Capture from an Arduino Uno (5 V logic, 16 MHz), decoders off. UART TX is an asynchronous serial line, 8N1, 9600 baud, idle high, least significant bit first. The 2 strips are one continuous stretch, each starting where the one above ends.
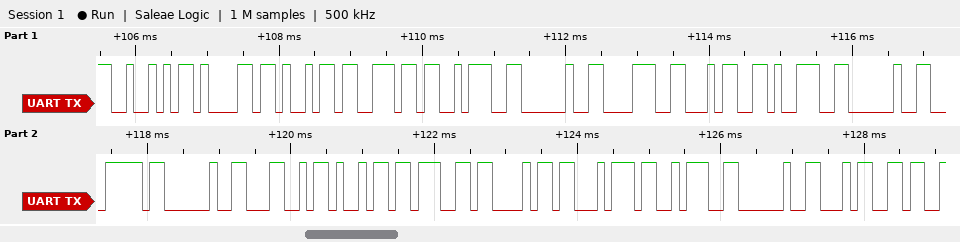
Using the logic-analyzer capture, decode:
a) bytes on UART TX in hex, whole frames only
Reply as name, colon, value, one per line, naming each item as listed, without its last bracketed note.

bytes on UART TX in hex, whole frames only: 52 61 69 6E 3A 20 38 34 39 20 7C 20 4C 69 67 68 74 3A 20 34
